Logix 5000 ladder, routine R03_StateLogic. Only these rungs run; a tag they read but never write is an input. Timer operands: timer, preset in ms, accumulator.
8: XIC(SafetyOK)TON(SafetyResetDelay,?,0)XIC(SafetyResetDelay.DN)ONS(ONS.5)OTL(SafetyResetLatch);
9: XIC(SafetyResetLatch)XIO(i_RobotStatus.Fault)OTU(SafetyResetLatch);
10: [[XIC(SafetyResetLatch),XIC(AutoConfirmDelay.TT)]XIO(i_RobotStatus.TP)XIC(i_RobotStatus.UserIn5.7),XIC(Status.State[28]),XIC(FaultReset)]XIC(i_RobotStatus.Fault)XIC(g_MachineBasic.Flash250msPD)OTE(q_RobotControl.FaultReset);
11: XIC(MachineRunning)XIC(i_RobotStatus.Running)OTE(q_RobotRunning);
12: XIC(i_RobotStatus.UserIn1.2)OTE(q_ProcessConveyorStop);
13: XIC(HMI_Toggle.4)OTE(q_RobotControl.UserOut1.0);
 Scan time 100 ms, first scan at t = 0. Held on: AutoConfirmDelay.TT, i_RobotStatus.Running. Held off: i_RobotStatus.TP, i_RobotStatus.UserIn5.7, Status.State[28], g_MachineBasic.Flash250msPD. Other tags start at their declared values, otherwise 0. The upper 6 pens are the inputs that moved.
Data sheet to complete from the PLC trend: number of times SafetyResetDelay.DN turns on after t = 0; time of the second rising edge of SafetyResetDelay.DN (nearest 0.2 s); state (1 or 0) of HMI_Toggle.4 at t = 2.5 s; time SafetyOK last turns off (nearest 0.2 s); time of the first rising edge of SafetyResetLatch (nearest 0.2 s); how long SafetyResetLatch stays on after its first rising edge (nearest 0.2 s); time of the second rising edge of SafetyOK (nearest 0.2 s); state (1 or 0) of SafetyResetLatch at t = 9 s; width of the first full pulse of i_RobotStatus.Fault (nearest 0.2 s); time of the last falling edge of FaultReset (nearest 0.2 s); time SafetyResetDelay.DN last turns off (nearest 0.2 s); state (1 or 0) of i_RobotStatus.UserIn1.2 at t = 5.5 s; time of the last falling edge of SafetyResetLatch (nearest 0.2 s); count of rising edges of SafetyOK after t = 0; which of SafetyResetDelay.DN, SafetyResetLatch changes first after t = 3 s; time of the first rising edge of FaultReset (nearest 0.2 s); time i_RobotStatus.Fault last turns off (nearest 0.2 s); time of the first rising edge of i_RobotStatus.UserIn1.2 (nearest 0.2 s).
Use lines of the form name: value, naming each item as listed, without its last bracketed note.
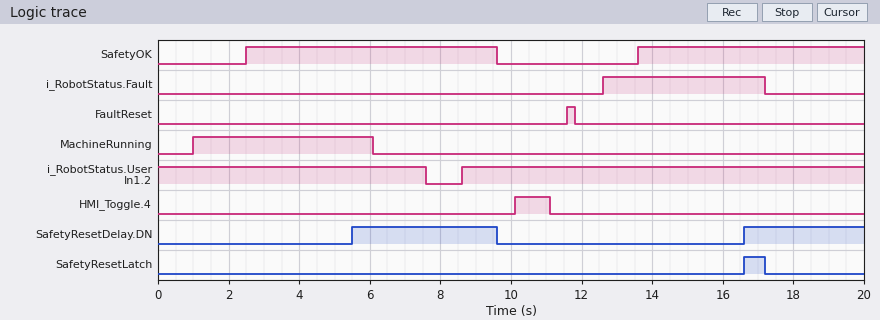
number of times SafetyResetDelay.DN turns on after t = 0: 2
time of the second rising edge of SafetyResetDelay.DN: 16.6 s
state (1 or 0) of HMI_Toggle.4 at t = 2.5 s: 0
time SafetyOK last turns off: 9.6 s
time of the first rising edge of SafetyResetLatch: 16.6 s
how long SafetyResetLatch stays on after its first rising edge: 0.6 s
time of the second rising edge of SafetyOK: 13.6 s
state (1 or 0) of SafetyResetLatch at t = 9 s: 0
width of the first full pulse of i_RobotStatus.Fault: 4.6 s
time of the last falling edge of FaultReset: 11.8 s
time SafetyResetDelay.DN last turns off: 9.6 s
state (1 or 0) of i_RobotStatus.UserIn1.2 at t = 5.5 s: 1
time of the last falling edge of SafetyResetLatch: 17.2 s
count of rising edges of SafetyOK after t = 0: 2
which of SafetyResetDelay.DN, SafetyResetLatch changes first after t = 3 s: SafetyResetDelay.DN
time of the first rising edge of FaultReset: 11.6 s
time i_RobotStatus.Fault last turns off: 17.2 s
time of the first rising edge of i_RobotStatus.UserIn1.2: 8.6 s
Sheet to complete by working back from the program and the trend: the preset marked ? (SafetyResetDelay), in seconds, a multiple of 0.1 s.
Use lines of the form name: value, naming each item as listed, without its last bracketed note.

the preset marked ? (SafetyResetDelay), in seconds, a multiple of 0.1 s: 3.0 s
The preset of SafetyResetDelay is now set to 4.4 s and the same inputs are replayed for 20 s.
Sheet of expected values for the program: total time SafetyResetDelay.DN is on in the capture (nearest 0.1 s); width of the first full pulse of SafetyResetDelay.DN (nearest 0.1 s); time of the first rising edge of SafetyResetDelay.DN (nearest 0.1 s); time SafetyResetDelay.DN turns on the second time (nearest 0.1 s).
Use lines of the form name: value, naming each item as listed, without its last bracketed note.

total time SafetyResetDelay.DN is on in the capture: 4.7 s
width of the first full pulse of SafetyResetDelay.DN: 2.7 s
time of the first rising edge of SafetyResetDelay.DN: 6.9 s
time SafetyResetDelay.DN turns on the second time: 18.0 s
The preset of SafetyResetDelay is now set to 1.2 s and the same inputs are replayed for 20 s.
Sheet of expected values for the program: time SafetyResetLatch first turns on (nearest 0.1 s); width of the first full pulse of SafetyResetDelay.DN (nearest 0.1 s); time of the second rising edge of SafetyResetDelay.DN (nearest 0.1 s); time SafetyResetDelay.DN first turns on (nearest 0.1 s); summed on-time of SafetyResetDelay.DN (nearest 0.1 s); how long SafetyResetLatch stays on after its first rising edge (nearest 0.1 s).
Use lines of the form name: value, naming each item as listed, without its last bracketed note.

time SafetyResetLatch first turns on: 14.8 s
width of the first full pulse of SafetyResetDelay.DN: 5.9 s
time of the second rising edge of SafetyResetDelay.DN: 14.8 s
time SafetyResetDelay.DN first turns on: 3.7 s
summed on-time of SafetyResetDelay.DN: 11.1 s
how long SafetyResetLatch stays on after its first rising edge: 2.4 s
